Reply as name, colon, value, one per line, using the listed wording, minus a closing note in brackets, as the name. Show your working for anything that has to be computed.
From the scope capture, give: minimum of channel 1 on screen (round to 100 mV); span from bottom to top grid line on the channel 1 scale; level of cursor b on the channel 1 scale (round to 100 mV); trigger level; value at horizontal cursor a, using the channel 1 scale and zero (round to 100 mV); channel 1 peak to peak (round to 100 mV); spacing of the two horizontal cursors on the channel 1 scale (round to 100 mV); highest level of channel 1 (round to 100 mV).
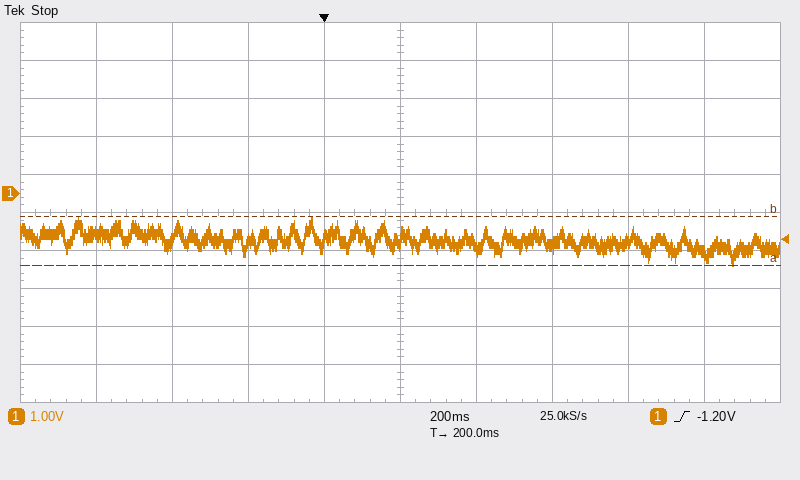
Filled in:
minimum of channel 1 on screen: -1.9 V
span from bottom to top grid line on the channel 1 scale: 10 V
level of cursor b on the channel 1 scale: -600 mV
trigger level: -1.20 V
value at horizontal cursor a, using the channel 1 scale and zero: -1.9 V
channel 1 peak to peak: -600 mV − (-1.9 V) = 1.3 V
spacing of the two horizontal cursors on the channel 1 scale: 1.3 V
highest level of channel 1: -600 mV
